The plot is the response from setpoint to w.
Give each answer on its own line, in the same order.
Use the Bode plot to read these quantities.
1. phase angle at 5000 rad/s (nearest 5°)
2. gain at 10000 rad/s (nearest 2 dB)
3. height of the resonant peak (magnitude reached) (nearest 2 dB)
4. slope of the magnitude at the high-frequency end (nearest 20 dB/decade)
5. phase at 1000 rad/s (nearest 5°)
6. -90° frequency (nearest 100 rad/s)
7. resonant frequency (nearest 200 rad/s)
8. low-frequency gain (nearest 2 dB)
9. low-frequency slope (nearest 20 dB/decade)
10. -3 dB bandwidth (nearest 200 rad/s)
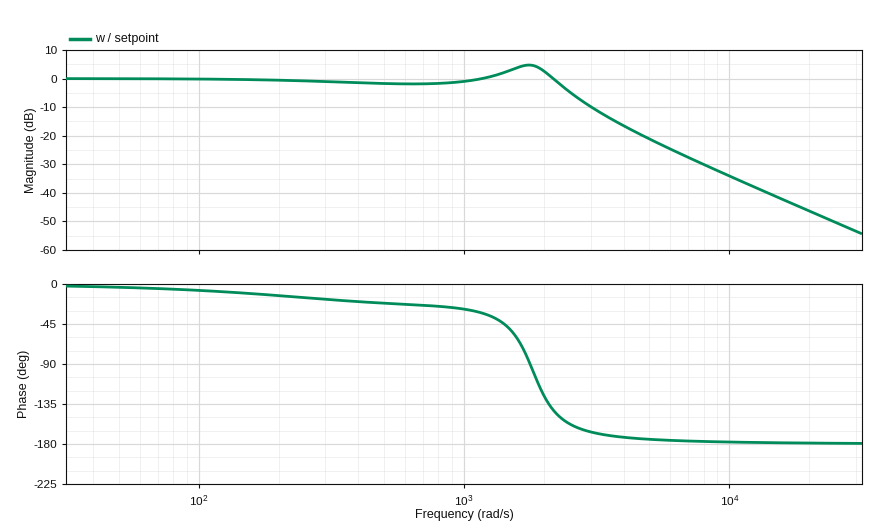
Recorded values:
-175°
-34 dB
4 dB
-40 dB/decade
-30°
1800 rad/s
1800 rad/s
0 dB
0 dB/decade
2400 rad/s
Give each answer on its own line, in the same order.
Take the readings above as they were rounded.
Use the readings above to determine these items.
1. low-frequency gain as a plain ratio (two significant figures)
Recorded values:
1.0
